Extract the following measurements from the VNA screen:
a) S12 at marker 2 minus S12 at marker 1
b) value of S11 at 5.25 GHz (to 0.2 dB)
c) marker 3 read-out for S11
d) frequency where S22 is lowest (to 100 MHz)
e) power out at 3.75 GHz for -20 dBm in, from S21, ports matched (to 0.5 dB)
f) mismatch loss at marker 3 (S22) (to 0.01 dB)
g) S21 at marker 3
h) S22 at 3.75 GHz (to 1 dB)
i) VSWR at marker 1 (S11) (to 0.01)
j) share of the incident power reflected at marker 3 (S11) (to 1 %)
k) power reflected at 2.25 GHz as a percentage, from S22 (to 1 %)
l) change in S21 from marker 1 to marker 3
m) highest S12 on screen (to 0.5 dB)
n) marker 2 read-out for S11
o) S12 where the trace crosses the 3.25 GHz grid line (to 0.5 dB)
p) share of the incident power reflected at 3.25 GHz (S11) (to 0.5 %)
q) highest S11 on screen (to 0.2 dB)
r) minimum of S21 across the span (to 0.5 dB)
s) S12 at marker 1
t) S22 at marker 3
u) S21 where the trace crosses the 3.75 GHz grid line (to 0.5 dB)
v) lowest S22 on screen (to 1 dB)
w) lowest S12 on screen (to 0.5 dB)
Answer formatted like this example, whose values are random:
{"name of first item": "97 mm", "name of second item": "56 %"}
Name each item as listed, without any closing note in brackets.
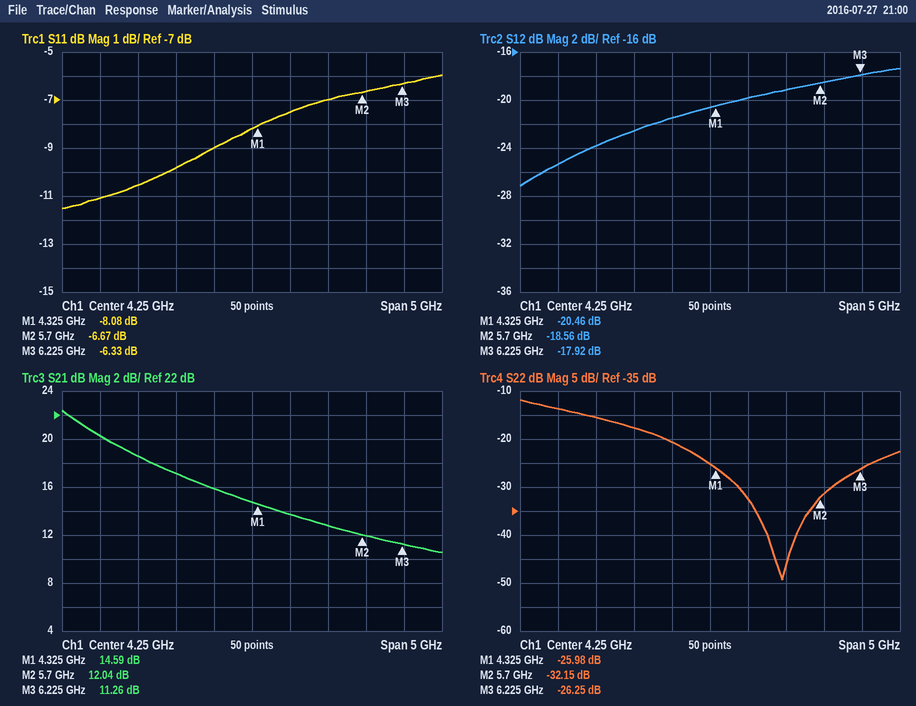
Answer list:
{"S12 at marker 2 minus S12 at marker 1": "1.90 dB", "value of S11 at 5.25 GHz": "-7.0 dB", "marker 3 read-out for S11": "-6.33 dB", "frequency where S22 is lowest": "5.2 GHz", "power out at 3.75 GHz for -20 dBm in, from S21, ports matched": "-4.0 dBm", "mismatch loss at marker 3 (S22)": "0.01 dB", "S21 at marker 3": "11.26 dB", "S22 at 3.75 GHz": "-21 dB", "VSWR at marker 1 (S11)": "2.30", "share of the incident power reflected at marker 3 (S11)": "23 %", "power reflected at 2.25 GHz as a percentage, from S22": "4 %", "change in S21 from marker 1 to marker 3": "-3.33 dB", "highest S12 on screen": "-17.5 dB", "marker 2 read-out for S11": "-6.67 dB", "S12 where the trace crosses the 3.25 GHz grid line": "-22.5 dB", "share of the incident power reflected at 3.25 GHz (S11)": "10.5 %", "highest S11 on screen": "-6.0 dB", "minimum of S21 across the span": "10.5 dB", "S12 at marker 1": "-20.46 dB", "S22 at marker 3": "-26.25 dB", "S21 where the trace crosses the 3.75 GHz grid line": "16.0 dB", "lowest S22 on screen": "-49 dB", "lowest S12 on screen": "-27.0 dB"}
